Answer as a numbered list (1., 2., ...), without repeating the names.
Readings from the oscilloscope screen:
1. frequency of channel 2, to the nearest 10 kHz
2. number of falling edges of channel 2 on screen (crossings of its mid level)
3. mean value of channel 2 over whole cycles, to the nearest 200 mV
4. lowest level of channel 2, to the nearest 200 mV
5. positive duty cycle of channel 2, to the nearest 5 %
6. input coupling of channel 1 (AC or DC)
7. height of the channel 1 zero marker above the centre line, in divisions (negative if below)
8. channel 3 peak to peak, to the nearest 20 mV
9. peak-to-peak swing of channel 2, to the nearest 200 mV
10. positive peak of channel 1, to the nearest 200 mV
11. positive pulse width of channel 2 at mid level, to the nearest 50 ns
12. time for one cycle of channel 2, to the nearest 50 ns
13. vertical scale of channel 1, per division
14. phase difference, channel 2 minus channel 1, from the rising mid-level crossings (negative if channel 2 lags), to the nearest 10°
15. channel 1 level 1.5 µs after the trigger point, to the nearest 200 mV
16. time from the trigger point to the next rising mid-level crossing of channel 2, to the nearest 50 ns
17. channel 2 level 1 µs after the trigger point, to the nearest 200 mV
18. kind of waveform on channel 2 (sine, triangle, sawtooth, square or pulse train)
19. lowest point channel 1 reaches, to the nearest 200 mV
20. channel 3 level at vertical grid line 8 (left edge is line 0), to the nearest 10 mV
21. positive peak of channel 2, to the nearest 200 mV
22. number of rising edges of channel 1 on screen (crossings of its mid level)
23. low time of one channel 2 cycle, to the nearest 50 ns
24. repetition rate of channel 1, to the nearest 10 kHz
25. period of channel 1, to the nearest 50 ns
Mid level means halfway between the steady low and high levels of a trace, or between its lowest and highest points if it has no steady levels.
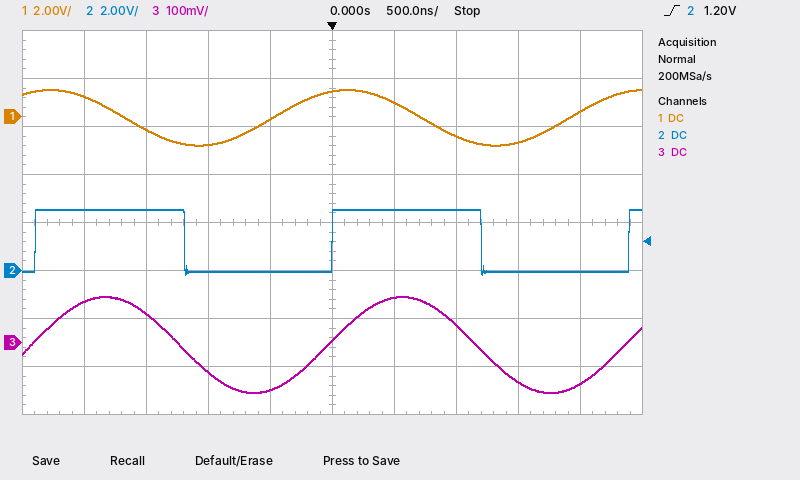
1. 420 kHz
2. 2
3. 1.2 V
4. -200 mV
5. 50 %
6. DC
7. +2.2 div
8. 200 mV
9. 2.8 V
10. 1.2 V
11. 1.20 µs
12. 2.40 µs
13. 2 V
14. -70°
15. -1.0 V
16. 2.40 µs
17. 2.6 V
18. square
19. -1.2 V
20. -80 mV
21. 2.6 V
22. 2
23. 1.20 µs
24. 420 kHz
25. 2.40 µs
